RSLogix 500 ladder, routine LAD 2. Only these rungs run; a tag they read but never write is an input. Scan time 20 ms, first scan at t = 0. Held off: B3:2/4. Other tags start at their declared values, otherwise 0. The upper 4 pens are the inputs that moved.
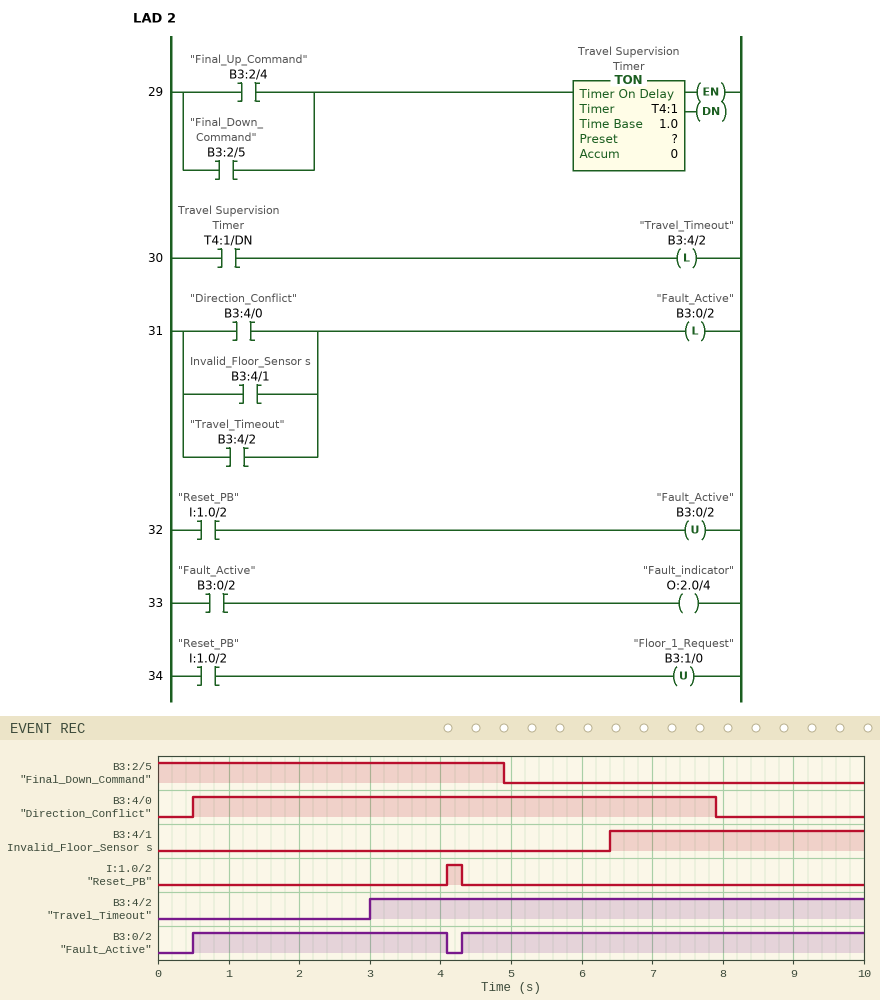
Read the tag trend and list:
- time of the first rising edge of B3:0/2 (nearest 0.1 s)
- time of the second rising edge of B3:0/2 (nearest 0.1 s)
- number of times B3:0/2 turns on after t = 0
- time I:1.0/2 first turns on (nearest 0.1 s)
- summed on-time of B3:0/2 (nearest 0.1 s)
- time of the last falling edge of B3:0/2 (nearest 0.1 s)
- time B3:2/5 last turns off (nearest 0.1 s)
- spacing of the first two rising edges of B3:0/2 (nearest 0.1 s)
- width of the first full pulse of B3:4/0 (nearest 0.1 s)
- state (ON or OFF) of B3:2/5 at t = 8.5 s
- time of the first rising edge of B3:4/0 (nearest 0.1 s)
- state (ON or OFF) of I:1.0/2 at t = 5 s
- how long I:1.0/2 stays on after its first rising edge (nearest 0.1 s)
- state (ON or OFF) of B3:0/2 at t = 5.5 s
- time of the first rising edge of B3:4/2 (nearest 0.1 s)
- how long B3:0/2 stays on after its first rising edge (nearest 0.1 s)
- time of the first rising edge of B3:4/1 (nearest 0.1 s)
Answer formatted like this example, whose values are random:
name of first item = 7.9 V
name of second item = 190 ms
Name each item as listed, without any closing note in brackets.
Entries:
time of the first rising edge of B3:0/2 = 0.5 s
time of the second rising edge of B3:0/2 = 4.3 s
number of times B3:0/2 turns on after t = 0 = 2
time I:1.0/2 first turns on = 4.1 s
summed on-time of B3:0/2 = 9.3 s
time of the last falling edge of B3:0/2 = 4.1 s
time B3:2/5 last turns off = 4.9 s
spacing of the first two rising edges of B3:0/2 = 3.8 s
width of the first full pulse of B3:4/0 = 7.4 s
state (ON or OFF) of B3:2/5 at t = 8.5 s = OFF
time of the first rising edge of B3:4/0 = 0.5 s
state (ON or OFF) of I:1.0/2 at t = 5 s = OFF
how long I:1.0/2 stays on after its first rising edge = 0.2 s
state (ON or OFF) of B3:0/2 at t = 5.5 s = ON
time of the first rising edge of B3:4/2 = 3.0 s
how long B3:0/2 stays on after its first rising edge = 3.6 s
time of the first rising edge of B3:4/1 = 6.4 s
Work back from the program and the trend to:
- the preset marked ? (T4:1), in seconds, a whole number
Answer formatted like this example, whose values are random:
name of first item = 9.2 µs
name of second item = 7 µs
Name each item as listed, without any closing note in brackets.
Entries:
the preset marked ? (T4:1), in seconds, a whole number = 3 s
